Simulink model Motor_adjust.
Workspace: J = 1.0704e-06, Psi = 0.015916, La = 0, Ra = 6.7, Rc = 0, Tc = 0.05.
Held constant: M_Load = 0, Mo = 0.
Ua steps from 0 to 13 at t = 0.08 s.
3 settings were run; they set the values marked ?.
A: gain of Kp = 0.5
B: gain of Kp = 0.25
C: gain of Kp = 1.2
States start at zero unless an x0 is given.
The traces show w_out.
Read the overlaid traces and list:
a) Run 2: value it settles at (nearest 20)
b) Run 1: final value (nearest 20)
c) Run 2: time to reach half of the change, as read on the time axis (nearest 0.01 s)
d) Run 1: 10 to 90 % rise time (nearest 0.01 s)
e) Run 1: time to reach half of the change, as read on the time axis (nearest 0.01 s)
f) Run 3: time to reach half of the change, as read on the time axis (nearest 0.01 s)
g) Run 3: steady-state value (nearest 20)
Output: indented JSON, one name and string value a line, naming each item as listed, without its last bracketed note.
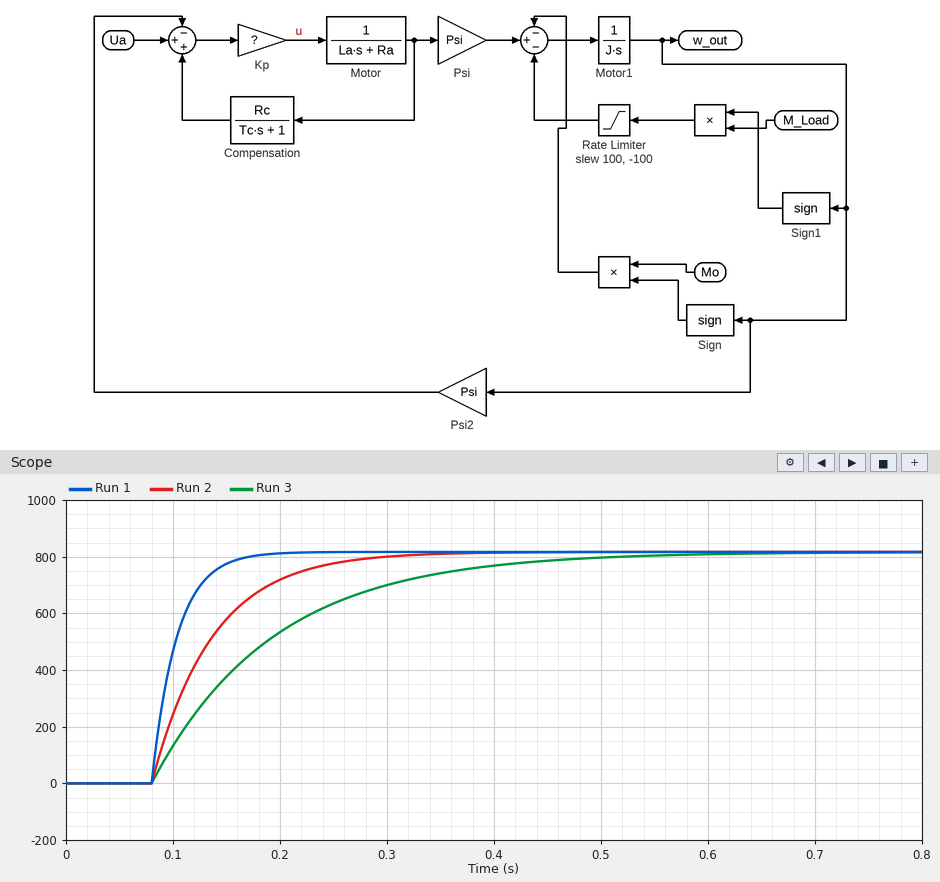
{
  "Run 2: value it settles at": "820",
  "Run 1: final value": "820",
  "Run 2: time to reach half of the change, as read on the time axis": "0.12 s",
  "Run 1: 10 to 90 % rise time": "0.05 s",
  "Run 1: time to reach half of the change, as read on the time axis": "0.10 s",
  "Run 3: time to reach half of the change, as read on the time axis": "0.16 s",
  "Run 3: steady-state value": "820"
}
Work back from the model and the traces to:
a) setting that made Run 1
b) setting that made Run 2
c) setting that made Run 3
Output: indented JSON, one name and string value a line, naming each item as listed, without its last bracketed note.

{
  "setting that made Run 1": "C",
  "setting that made Run 2": "A",
  "setting that made Run 3": "B"
}
